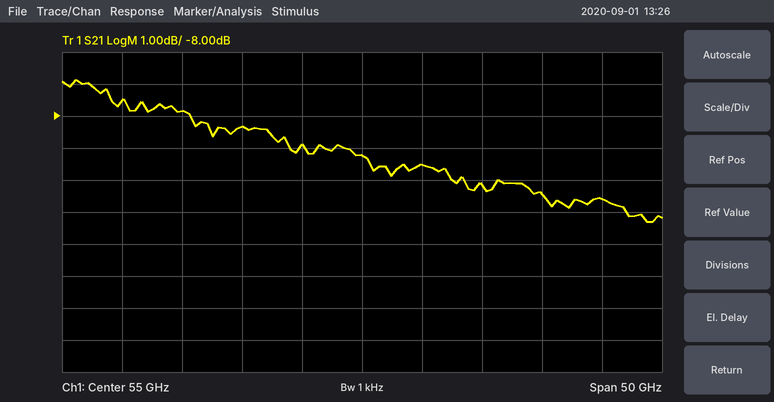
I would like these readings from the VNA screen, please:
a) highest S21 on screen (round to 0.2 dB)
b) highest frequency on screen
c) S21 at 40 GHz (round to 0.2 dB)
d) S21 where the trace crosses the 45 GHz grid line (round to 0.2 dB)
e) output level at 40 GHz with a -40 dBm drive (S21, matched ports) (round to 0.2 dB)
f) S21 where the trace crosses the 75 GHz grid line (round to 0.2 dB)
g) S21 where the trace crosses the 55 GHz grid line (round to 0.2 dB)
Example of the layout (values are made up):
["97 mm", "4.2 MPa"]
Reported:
["-6.8 dB", "80 GHz", "-7.8 dB", "-8.4 dB", "-47.8 dBm", "-10.6 dB", "-9.2 dB"]
